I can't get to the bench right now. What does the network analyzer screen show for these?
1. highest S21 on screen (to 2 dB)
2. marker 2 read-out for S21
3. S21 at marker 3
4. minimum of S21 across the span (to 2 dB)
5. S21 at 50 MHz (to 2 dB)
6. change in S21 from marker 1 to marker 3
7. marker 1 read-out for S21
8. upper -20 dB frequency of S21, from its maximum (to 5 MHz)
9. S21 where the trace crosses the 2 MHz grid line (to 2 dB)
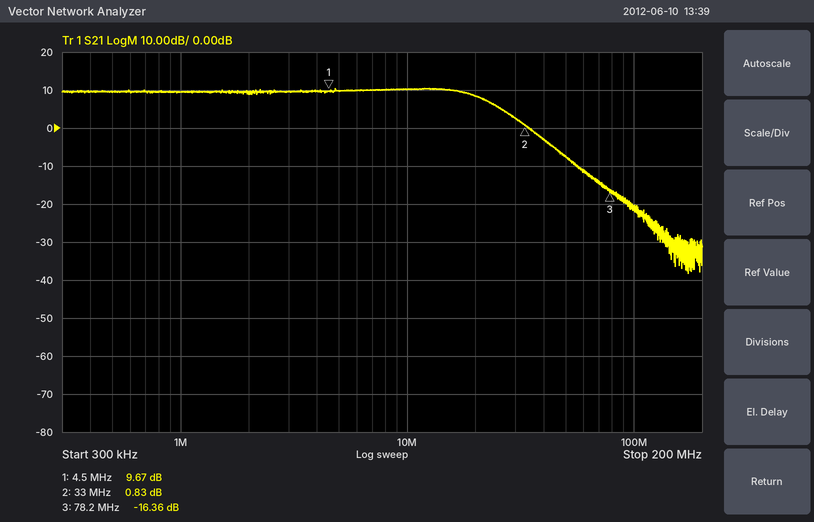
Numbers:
10 dB
0.83 dB
-16.36 dB
-38 dB
-8 dB
-26.03 dB
9.67 dB
55 MHz
10 dB
